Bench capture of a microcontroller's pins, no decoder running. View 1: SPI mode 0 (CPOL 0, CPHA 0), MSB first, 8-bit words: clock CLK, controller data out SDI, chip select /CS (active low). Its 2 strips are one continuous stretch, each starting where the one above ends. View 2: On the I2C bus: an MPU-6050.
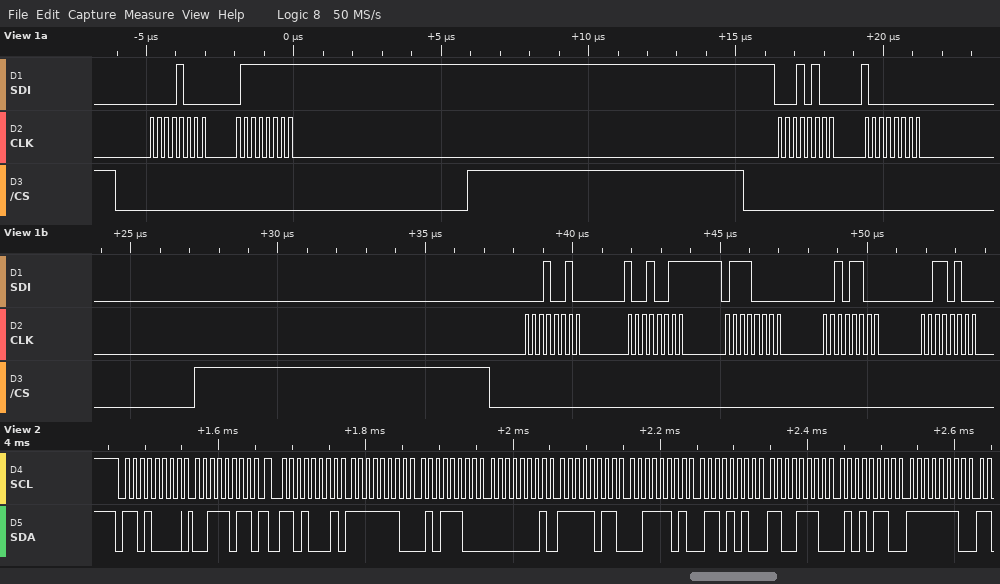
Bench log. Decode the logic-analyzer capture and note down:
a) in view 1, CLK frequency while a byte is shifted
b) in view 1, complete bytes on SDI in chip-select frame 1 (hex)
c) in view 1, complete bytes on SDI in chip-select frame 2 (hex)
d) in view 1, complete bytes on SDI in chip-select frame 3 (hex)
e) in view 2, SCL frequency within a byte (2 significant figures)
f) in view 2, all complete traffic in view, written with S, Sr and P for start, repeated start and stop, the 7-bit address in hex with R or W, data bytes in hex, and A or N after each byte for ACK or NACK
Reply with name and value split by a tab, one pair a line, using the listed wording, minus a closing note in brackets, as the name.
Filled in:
in view 1, CLK frequency while a byte is shifted	4 MHz
in view 1, complete bytes on SDI in chip-select frame 1	08 7F
in view 1, complete bytes on SDI in chip-select frame 2	14 80
in view 1, complete bytes on SDI in chip-select frame 3	12 93 70 2C 34
in view 2, SCL frequency within a byte	100 kHz
in view 2, all complete traffic in view, written with S, Sr and P for start, repeated start and stop, the 7-bit address in hex with R or W, data bytes in hex, and A or N after each byte for ACK or NACK	S 68W A 3B A Sr 68R A FE A 5C A 01 A FB A 3D A 6A A CE A 56 A FE A
